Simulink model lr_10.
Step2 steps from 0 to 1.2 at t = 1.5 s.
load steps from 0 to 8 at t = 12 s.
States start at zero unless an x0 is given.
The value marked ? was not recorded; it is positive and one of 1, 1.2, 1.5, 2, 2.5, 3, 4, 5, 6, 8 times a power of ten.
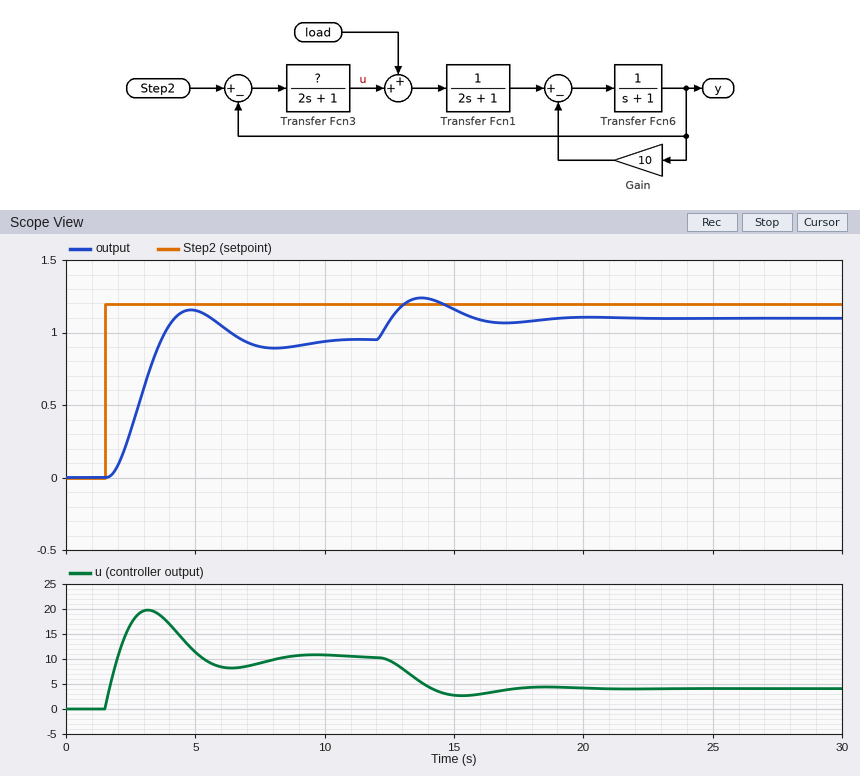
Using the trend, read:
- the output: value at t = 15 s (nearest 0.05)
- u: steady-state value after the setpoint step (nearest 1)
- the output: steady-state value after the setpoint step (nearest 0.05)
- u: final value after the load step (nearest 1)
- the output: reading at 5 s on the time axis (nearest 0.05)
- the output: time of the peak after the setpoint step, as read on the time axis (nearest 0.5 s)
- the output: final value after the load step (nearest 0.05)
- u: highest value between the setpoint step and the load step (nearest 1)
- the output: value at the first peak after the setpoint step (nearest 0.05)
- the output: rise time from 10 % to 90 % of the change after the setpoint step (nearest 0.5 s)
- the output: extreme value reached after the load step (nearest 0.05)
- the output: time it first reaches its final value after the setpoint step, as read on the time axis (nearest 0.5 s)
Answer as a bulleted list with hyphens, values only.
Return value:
- 1.15
- 10
- 0.95
- 4
- 1.15
- 5.0 s
- 1.10
- 20
- 1.15
- 1.5 s
- 1.25
- 3.5 s
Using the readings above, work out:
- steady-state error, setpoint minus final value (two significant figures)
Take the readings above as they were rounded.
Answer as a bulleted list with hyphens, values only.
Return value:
- 0.25
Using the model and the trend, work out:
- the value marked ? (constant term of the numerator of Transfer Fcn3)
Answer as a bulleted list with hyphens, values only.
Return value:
- 40
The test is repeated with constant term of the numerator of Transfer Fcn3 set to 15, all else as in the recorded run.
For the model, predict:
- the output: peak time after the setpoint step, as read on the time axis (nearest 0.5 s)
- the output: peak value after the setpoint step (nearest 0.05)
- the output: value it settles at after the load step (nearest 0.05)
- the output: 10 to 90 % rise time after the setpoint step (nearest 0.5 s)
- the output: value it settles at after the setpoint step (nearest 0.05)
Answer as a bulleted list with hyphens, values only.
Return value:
- 7.0 s
- 0.75
- 1.00
- 2.5 s
- 0.70
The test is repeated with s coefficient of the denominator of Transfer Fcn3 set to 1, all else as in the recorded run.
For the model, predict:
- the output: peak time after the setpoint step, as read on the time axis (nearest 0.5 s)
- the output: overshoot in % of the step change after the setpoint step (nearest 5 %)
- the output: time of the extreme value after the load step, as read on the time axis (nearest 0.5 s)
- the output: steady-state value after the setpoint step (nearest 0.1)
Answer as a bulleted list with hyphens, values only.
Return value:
- 4.0 s
- 20 %
- 13.5 s
- 0.9
